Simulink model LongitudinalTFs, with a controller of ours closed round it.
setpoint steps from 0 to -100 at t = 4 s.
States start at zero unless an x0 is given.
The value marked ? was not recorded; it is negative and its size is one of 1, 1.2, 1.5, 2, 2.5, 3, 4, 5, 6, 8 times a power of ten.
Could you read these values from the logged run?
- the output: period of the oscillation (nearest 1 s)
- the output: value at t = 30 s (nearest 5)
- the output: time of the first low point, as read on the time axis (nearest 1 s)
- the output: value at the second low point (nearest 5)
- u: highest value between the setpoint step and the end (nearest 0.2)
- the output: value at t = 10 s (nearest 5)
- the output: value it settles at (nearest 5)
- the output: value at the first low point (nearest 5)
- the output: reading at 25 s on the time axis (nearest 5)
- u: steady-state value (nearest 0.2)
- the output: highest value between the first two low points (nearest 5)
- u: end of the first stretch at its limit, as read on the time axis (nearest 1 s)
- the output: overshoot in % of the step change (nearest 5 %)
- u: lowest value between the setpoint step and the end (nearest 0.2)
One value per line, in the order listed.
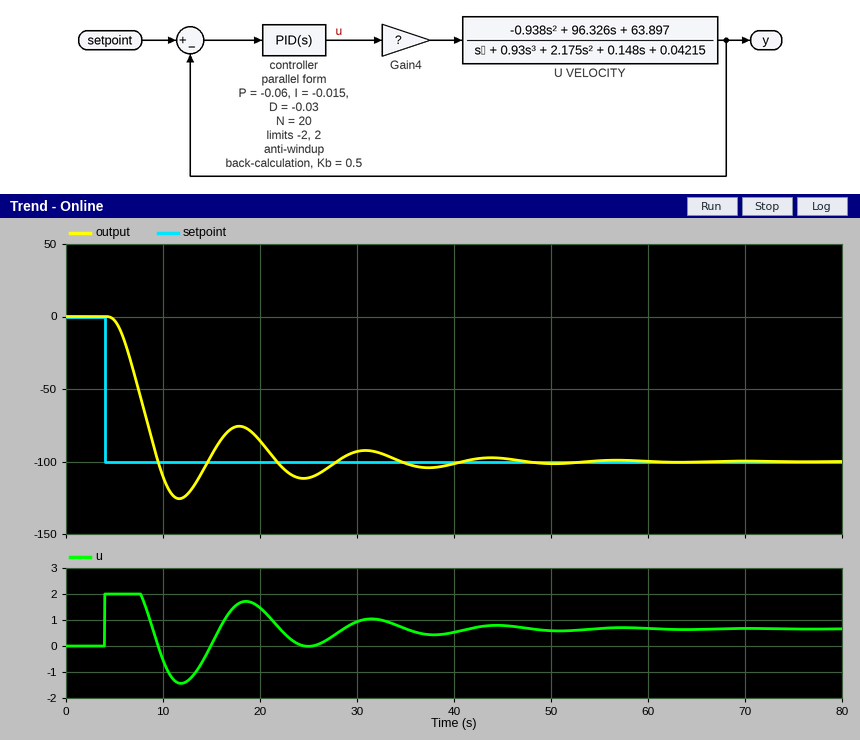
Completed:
13 s
-95
12 s
-110
2.0
-110
-100
-125
-110
0.6
-75
8 s
25 %
-1.4
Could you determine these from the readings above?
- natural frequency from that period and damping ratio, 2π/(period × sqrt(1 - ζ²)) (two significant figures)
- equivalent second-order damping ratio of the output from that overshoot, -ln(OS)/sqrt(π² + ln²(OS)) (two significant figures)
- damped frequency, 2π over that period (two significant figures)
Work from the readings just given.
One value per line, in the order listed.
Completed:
0.53 rad/s
0.40
0.48 rad/s
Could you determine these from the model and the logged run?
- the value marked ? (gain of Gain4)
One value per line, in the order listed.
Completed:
-0.1
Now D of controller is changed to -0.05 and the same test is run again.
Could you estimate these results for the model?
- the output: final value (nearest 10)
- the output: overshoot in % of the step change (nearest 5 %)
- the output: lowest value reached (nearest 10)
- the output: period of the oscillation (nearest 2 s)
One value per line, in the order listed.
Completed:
-100
20 %
-120
14 s
